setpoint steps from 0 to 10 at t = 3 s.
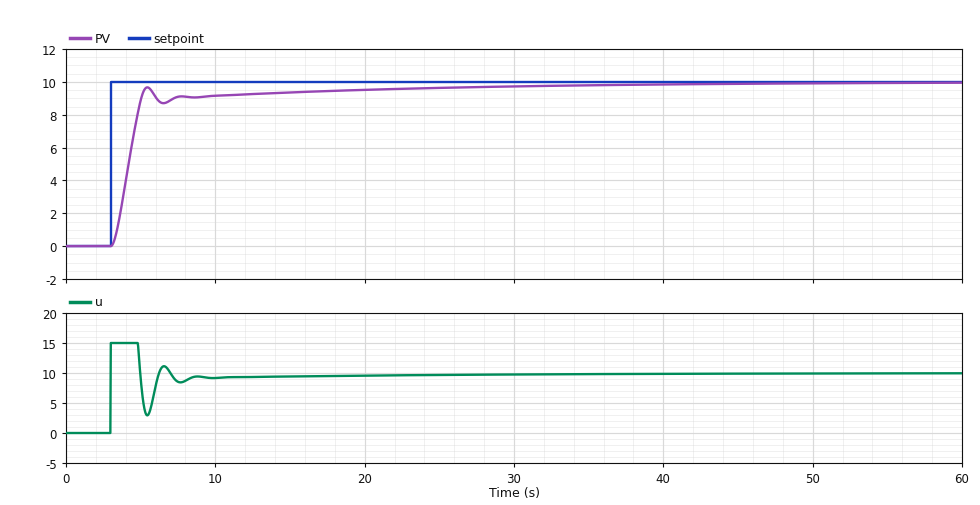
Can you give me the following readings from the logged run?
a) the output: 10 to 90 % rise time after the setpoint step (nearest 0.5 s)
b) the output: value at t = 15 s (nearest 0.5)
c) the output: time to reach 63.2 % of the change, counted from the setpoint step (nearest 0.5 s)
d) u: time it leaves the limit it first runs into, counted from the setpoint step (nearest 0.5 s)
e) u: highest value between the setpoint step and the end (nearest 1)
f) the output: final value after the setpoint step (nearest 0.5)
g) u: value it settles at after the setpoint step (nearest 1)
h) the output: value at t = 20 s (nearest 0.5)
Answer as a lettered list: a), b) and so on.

a) 1.5 s
b) 9.5
c) 1.5 s
d) 2.0 s
e) 15
f) 10.0
g) 10
h) 9.5
